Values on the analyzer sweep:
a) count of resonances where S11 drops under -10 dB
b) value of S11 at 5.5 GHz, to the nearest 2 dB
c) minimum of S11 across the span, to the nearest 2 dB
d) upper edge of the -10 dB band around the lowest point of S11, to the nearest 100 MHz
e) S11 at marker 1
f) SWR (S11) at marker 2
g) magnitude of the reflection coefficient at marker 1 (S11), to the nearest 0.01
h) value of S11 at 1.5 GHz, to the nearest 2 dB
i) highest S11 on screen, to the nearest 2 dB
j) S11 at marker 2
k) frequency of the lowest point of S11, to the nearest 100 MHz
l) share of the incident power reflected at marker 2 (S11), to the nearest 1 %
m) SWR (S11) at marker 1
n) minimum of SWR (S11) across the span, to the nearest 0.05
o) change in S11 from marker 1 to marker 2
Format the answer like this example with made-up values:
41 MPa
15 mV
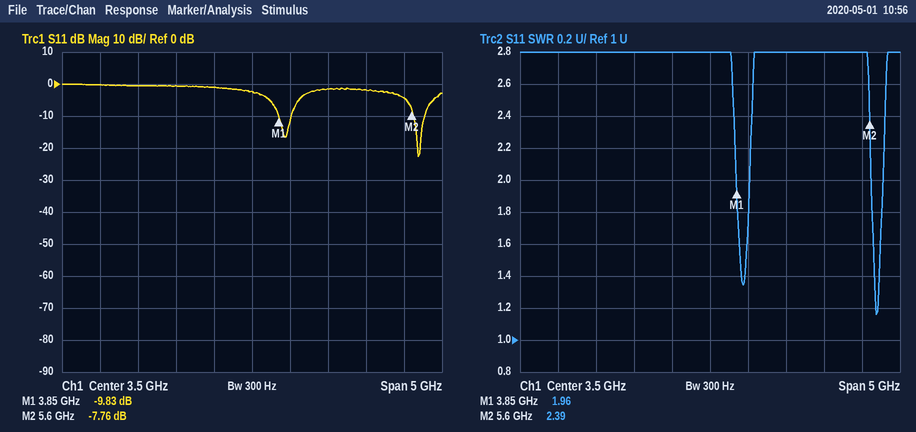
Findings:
2
-4 dB
-22 dB
5.8 GHz
-9.83 dB
2.39
0.32
0 dB
0 dB
-7.76 dB
5.7 GHz
17 %
1.96
1.15
2.07 dB
